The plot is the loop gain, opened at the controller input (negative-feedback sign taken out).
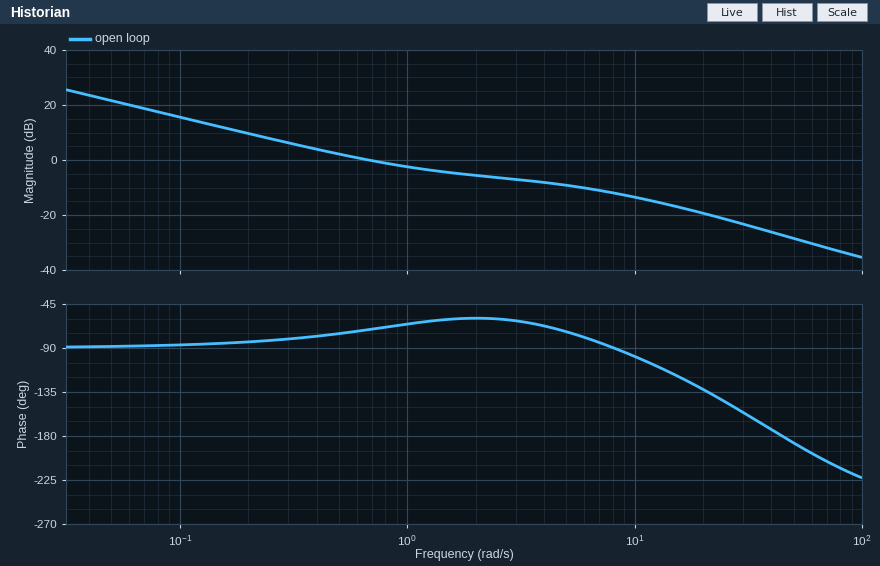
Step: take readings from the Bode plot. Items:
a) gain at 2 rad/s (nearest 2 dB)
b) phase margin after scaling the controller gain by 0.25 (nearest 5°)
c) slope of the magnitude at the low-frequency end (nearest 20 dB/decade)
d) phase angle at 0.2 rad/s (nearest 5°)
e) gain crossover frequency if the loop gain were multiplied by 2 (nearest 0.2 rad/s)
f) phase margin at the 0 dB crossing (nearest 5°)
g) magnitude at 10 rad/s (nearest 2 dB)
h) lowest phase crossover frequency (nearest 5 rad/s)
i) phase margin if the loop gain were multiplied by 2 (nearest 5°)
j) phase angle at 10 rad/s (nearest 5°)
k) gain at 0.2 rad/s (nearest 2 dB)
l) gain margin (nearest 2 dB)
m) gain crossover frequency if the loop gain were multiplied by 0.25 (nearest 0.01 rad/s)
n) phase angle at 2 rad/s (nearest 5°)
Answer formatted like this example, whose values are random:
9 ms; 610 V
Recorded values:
-6 dB; 95°; -20 dB/decade; -85°; 2.2 rad/s; 110°; -14 dB; 45 rad/s; 120°; -100°; 10 dB; 28 dB; 0.15 rad/s; -60°
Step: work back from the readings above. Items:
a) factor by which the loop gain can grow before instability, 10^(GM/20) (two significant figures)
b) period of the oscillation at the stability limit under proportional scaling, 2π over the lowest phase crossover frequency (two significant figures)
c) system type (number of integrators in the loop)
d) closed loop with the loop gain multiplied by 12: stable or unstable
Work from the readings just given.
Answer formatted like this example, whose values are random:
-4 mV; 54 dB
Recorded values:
25; 0.14 s; 1; stable
